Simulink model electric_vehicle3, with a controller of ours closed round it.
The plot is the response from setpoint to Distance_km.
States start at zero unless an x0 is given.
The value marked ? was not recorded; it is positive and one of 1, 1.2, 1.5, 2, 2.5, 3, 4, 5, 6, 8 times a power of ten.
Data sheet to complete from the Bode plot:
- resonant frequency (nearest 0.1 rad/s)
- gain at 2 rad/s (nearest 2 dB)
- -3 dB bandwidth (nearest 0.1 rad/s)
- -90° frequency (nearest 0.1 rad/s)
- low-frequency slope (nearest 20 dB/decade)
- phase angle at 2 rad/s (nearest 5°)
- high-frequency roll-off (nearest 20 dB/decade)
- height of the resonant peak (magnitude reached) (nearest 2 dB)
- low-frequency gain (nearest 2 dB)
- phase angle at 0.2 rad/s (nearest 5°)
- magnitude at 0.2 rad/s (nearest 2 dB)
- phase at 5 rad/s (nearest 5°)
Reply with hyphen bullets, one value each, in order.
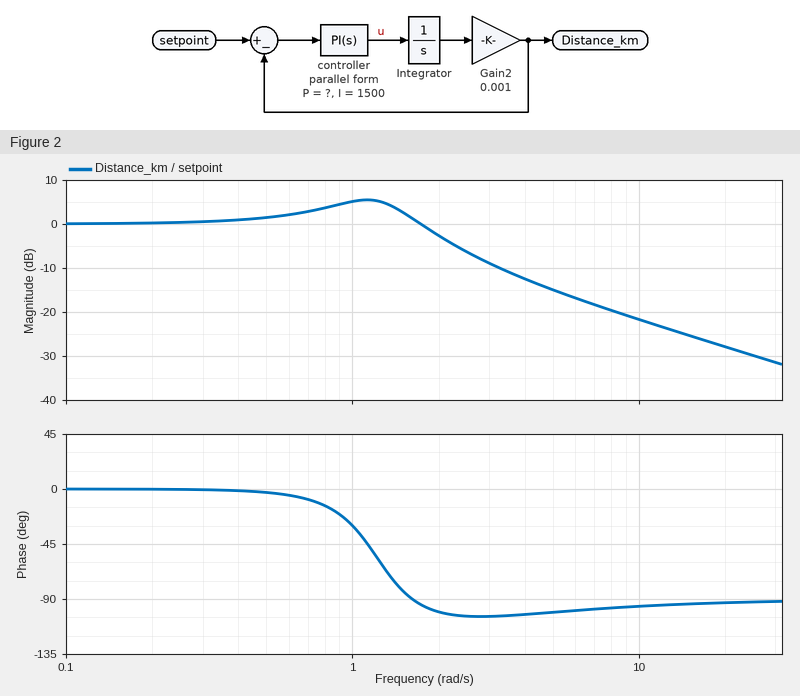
- 1.1 rad/s
- -2 dB
- 2.0 rad/s
- 1.6 rad/s
- 0 dB/decade
- -100°
- -20 dB/decade
- 6 dB
- 0 dB
- 0°
- 0 dB
- -100°
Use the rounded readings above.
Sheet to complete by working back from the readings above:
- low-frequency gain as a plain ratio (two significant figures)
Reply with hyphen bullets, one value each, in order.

- 1.0
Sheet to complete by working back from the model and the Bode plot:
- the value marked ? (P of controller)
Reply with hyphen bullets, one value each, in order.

- 800
